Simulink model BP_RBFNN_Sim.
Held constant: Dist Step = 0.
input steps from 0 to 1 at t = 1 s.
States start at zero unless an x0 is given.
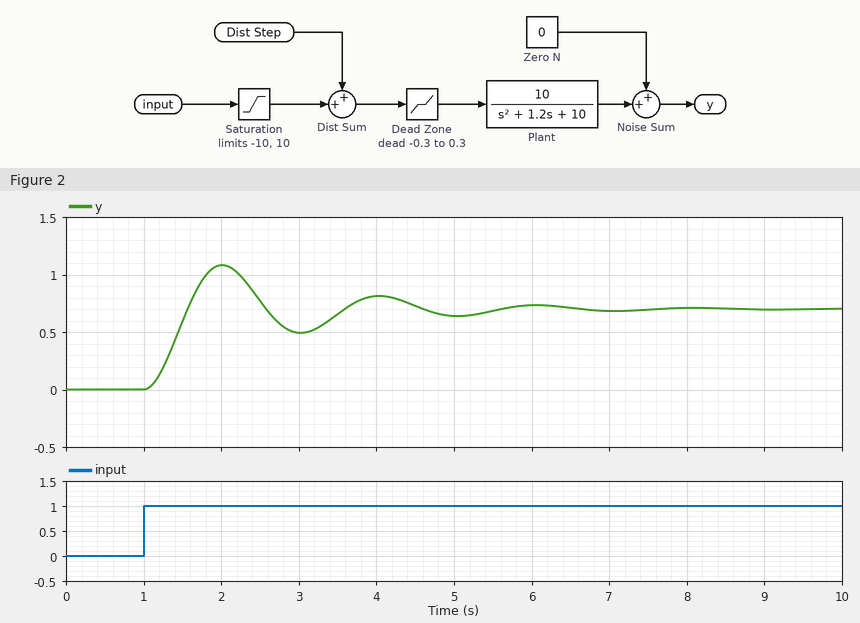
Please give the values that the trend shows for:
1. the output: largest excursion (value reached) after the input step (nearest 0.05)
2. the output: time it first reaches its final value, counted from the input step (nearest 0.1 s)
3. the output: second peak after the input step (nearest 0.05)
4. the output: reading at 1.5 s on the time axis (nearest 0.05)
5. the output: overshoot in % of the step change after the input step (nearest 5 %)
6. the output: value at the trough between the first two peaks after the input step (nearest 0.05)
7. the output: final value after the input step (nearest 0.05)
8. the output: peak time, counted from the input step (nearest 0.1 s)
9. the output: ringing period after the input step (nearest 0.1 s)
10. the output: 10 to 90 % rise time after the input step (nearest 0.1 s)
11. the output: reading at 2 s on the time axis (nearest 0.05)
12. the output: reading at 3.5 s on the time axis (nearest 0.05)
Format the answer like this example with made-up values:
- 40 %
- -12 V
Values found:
- 1.10
- 0.6 s
- 0.80
- 0.60
- 55 %
- 0.50
- 0.70
- 1.0 s
- 2.0 s
- 0.4 s
- 1.10
- 0.65
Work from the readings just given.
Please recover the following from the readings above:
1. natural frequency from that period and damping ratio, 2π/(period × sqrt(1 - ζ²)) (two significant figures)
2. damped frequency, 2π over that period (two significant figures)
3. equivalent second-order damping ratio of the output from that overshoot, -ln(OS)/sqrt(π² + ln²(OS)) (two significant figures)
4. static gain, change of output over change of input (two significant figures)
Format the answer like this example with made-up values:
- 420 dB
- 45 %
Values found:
- 3.2 rad/s
- 3.1 rad/s
- 0.19
- 0.70
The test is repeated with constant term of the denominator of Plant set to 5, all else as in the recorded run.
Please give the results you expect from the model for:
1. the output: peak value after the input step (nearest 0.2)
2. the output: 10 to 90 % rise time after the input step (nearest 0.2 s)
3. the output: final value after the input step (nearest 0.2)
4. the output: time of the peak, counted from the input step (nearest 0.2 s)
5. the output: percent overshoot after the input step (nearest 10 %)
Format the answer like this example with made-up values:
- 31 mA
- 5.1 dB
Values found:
- 2.0
- 0.6 s
- 1.4
- 1.4 s
- 40 %
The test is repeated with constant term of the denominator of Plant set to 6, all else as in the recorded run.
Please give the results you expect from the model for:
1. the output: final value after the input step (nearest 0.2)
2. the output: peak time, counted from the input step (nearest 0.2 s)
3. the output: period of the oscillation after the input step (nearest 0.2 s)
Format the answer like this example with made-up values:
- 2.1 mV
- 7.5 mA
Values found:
- 1.2
- 1.4 s
- 2.6 s
